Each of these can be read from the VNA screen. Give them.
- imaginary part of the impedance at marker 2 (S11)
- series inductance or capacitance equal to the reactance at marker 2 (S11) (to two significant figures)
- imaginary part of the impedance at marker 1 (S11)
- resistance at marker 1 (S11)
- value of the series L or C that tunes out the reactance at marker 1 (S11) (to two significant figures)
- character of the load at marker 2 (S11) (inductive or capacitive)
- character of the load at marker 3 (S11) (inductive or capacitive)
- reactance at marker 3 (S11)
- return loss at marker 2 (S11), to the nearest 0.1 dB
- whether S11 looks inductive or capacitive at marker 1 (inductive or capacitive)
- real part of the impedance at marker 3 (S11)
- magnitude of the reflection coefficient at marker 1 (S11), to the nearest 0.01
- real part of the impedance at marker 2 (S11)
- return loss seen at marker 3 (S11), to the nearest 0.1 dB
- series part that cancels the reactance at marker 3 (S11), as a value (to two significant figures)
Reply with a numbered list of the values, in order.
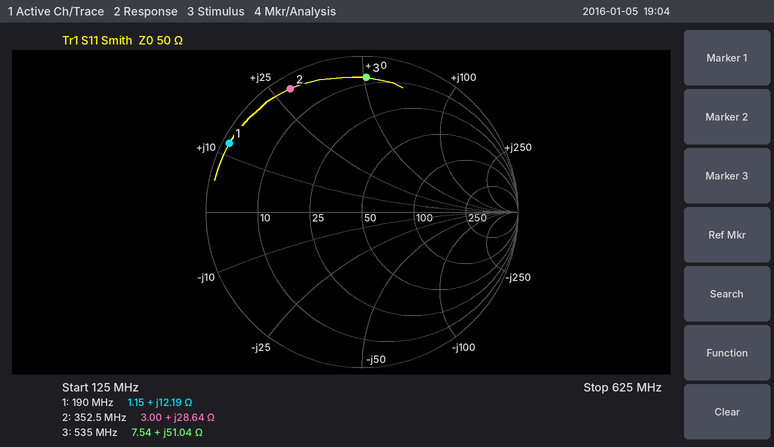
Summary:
1. +28.64 Ω
2. 13 nH
3. +12.19 Ω
4. 1.15 Ω
5. 69 pF
6. inductive
7. inductive
8. +51.04 Ω
9. 0.8 dB
10. inductive
11. 7.54 Ω
12. 0.96
13. 3.00 Ω
14. 1.3 dB
15. 5.8 pF
